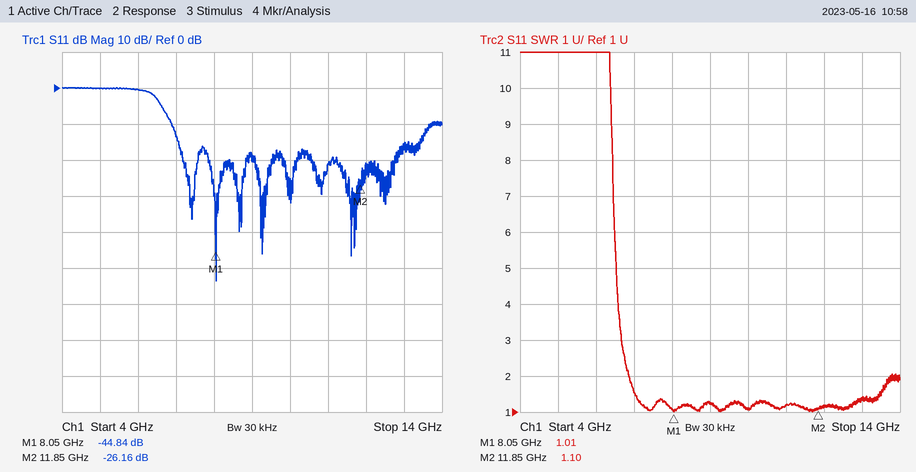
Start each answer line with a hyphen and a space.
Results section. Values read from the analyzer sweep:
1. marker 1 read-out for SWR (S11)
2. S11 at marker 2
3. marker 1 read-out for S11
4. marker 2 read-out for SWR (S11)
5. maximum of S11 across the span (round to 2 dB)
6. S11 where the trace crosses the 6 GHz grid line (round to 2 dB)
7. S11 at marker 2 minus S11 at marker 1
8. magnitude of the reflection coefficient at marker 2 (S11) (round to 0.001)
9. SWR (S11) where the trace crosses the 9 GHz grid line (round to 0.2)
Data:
- 1.01
- -26.16 dB
- -44.84 dB
- 1.10
- 0 dB
- 0 dB
- 18.68 dB
- 0.049
- 1.2
